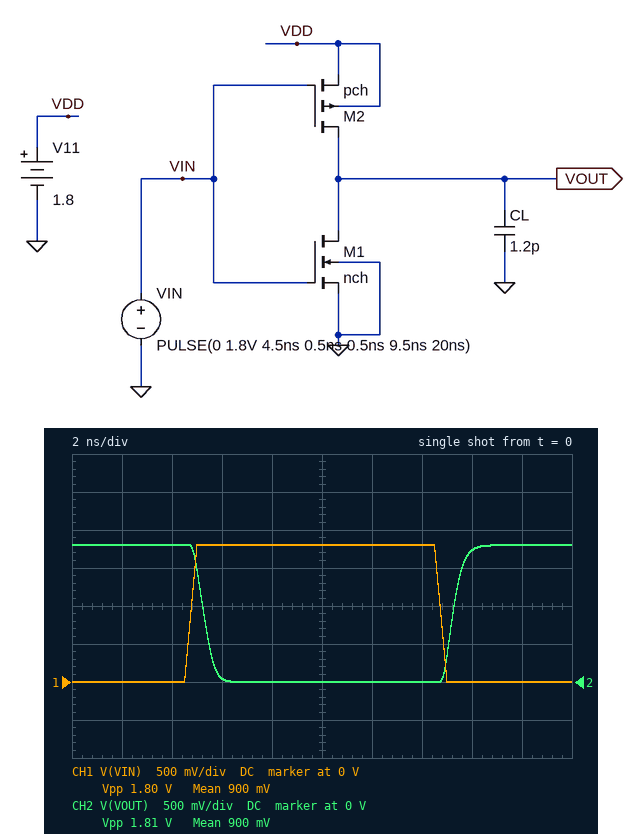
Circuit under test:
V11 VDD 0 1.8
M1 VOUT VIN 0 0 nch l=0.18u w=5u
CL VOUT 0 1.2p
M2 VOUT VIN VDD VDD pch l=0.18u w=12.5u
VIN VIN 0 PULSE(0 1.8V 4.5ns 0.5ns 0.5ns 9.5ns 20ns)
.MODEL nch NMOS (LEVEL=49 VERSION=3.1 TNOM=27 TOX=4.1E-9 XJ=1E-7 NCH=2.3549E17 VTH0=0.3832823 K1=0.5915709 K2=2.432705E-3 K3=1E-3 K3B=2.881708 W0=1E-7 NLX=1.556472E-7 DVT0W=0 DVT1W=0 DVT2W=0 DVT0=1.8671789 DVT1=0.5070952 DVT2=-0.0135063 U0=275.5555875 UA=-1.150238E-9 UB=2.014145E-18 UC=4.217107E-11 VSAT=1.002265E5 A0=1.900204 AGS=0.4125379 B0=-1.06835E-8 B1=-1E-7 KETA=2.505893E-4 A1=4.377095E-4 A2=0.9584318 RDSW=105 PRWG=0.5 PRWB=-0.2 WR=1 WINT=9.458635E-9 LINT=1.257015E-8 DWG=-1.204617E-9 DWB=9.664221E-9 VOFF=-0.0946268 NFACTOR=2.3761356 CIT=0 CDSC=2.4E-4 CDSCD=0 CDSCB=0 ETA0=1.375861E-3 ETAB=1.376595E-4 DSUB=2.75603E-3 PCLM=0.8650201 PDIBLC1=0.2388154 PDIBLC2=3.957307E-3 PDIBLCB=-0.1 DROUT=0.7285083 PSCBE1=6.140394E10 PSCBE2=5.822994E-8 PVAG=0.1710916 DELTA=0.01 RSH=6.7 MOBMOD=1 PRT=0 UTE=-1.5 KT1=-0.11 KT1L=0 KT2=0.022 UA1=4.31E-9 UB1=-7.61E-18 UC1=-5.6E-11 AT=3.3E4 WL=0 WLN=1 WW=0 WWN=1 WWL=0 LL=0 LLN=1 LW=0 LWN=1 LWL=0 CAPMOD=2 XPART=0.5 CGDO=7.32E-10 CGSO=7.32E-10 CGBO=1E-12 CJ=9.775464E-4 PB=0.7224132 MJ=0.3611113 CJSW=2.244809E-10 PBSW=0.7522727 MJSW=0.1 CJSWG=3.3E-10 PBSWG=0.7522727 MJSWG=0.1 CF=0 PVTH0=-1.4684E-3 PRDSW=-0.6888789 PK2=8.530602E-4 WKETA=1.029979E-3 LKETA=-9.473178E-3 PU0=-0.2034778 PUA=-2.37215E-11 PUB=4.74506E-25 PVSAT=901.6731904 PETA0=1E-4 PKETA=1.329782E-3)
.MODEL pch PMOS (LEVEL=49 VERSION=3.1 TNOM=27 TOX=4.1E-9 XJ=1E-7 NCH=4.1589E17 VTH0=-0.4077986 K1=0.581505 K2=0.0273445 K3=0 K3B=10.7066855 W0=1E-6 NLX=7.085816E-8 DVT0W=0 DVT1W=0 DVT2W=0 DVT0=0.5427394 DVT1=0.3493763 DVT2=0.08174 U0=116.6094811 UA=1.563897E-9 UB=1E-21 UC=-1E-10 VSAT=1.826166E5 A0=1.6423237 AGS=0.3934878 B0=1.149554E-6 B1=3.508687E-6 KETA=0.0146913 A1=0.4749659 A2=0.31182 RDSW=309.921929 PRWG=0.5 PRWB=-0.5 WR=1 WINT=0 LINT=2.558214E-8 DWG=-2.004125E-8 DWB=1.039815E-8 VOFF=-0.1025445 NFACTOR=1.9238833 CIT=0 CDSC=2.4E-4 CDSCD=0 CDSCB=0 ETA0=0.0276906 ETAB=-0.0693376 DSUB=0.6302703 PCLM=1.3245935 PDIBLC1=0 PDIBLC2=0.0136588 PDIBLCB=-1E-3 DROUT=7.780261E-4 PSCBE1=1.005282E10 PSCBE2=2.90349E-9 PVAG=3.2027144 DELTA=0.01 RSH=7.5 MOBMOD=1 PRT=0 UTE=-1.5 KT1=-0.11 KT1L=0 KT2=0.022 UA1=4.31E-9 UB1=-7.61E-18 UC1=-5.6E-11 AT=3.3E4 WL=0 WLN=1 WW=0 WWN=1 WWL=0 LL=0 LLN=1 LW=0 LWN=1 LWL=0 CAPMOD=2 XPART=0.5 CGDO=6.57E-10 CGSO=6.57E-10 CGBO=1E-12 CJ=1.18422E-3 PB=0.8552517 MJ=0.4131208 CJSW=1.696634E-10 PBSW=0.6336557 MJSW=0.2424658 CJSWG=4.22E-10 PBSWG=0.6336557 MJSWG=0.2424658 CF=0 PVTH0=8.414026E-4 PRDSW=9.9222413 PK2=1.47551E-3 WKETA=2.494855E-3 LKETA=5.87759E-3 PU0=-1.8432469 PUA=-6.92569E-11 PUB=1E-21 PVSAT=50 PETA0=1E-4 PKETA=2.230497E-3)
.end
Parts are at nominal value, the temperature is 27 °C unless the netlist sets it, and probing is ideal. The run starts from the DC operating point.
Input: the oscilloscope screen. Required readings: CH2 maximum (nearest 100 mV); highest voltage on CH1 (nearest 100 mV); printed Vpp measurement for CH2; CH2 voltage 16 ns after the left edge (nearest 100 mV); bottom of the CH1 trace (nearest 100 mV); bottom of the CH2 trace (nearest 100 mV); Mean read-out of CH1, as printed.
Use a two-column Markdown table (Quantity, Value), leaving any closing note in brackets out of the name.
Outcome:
| Quantity | Value |
|---|---|
| CH2 maximum | 1.8 V |
| highest voltage on CH1 | 1.8 V |
| printed Vpp measurement for CH2 | 1.81 V |
| CH2 voltage 16 ns after the left edge | 1.7 V |
| bottom of the CH1 trace | 0 V |
| bottom of the CH2 trace | 0 V |
| Mean read-out of CH1, as printed | 900 mV |
